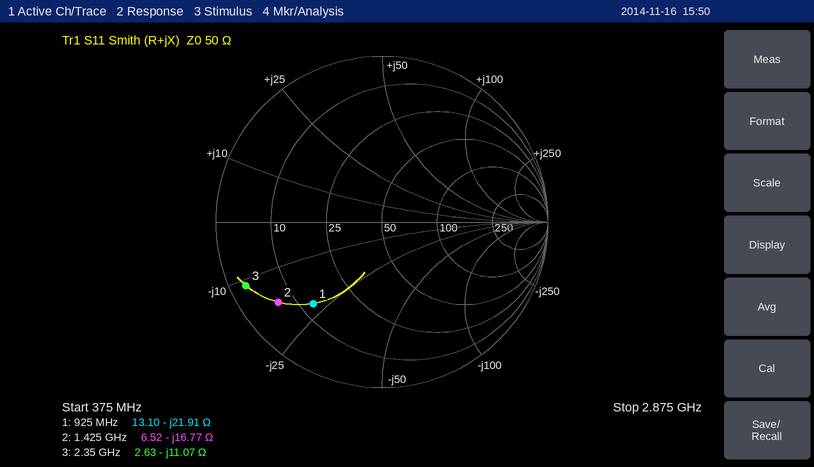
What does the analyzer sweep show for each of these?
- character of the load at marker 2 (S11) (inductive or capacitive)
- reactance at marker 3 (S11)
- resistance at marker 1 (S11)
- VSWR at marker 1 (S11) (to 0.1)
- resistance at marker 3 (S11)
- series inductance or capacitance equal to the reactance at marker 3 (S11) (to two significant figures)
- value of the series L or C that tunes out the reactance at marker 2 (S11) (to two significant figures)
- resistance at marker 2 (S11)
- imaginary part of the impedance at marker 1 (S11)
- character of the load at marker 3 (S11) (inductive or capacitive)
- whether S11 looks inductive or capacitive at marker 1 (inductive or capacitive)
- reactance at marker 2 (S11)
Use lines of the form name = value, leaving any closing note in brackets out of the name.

character of the load at marker 2 (S11) = capacitive
reactance at marker 3 = -11.07 Ω
resistance at marker 1 = 13.10 Ω
VSWR at marker 1 (S11) = 4.6
resistance at marker 3 = 2.63 Ω
series inductance or capacitance equal to the reactance at marker 3 (S11) = 6.1 pF
value of the series L or C that tunes out the reactance at marker 2 (S11) = 1.9 nH
resistance at marker 2 = 6.52 Ω
imaginary part of the impedance at marker 1 = -21.91 Ω
character of the load at marker 3 (S11) = capacitive
whether S11 looks inductive or capacitive at marker 1 = capacitive
reactance at marker 2 = -16.77 Ω
